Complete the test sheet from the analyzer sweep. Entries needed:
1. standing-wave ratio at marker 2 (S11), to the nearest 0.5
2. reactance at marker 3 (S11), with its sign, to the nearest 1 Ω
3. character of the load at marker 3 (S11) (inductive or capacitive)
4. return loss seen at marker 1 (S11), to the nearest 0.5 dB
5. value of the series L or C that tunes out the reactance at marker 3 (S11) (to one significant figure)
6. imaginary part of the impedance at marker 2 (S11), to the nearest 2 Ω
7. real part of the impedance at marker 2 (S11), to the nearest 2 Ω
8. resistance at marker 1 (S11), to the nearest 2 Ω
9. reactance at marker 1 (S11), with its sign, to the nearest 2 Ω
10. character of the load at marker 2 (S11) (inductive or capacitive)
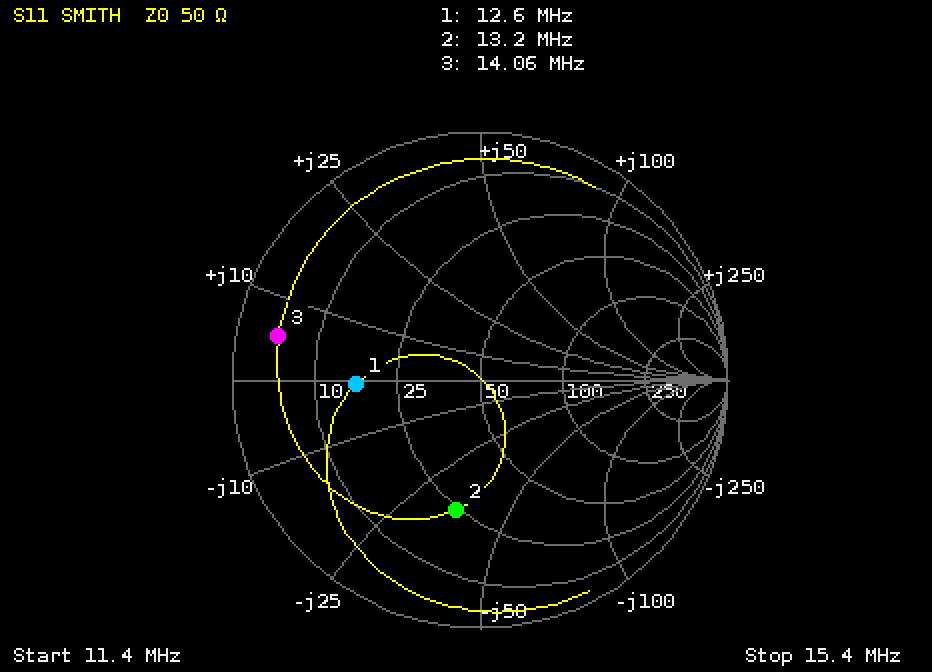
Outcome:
3.5
+5 Ω
inductive
6.0 dB
2 nF
-36 Ω
24 Ω
16 Ω
0 Ω
capacitive
